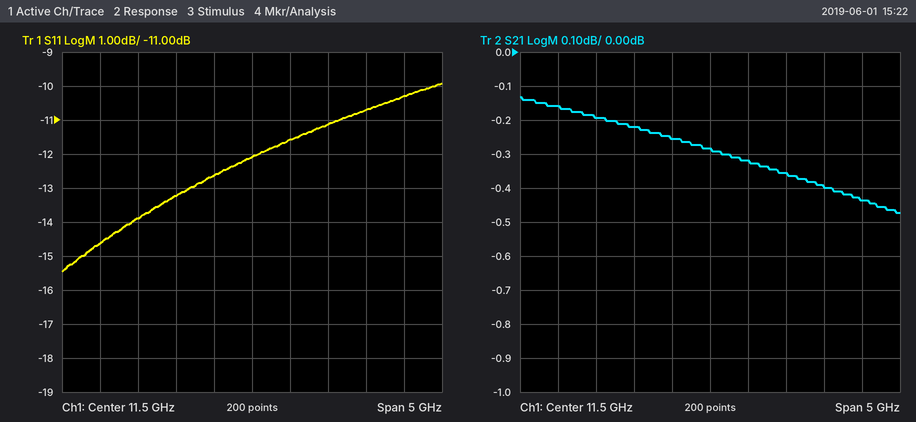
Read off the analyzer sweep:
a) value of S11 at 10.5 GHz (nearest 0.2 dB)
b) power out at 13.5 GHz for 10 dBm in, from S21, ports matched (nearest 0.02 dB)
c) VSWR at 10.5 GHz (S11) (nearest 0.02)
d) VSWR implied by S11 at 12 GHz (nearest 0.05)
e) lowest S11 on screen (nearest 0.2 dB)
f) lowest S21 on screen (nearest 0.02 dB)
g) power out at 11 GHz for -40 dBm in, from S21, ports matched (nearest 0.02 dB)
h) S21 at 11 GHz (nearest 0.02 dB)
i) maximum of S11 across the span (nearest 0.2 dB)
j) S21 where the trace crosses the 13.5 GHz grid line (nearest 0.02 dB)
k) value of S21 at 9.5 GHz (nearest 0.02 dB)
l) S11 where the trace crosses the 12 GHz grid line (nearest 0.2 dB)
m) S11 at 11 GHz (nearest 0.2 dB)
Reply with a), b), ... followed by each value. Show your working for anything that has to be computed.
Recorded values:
a) -13.2 dB
b) 10 dBm + (-0.44 dB) = 9.56 dBm
c) |Γ| = 10^(-13.2/20) = 0.2188; VSWR = (1 + 0.2188)/(1 − 0.2188) ≈ 1.56
d) |Γ| = 10^(-11.6/20) = 0.2630; VSWR = (1 + 0.2630)/(1 − 0.2630) ≈ 1.71, so 1.70 to the nearest 0.05
e) -15.4 dB
f) -0.48 dB
g) -40 dBm + (-0.26 dB) = -40.26 dBm
h) -0.26 dB
i) -10.0 dB
j) -0.44 dB
k) -0.16 dB
l) -11.6 dB
m) -12.6 dB
